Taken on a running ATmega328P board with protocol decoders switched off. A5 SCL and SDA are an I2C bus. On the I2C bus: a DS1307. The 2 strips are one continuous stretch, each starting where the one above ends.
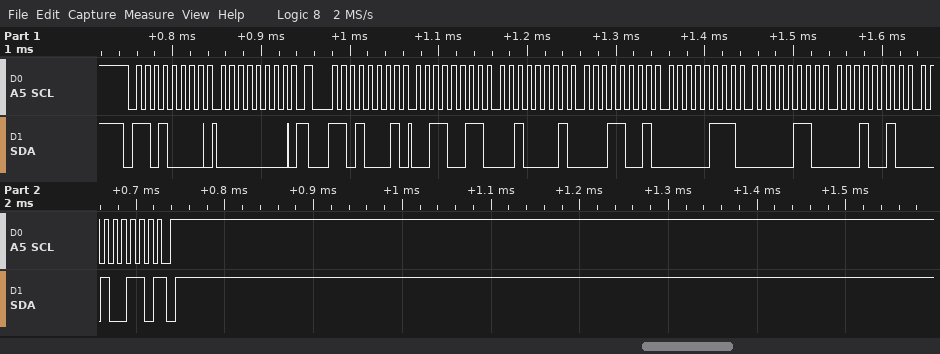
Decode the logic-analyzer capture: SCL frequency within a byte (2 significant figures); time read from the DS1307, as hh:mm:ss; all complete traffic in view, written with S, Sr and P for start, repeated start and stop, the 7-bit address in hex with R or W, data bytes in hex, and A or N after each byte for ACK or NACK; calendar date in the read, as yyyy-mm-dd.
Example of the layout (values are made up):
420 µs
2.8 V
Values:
100 kHz
19:21:33
S 68W A 00 A Sr 68R A 33 A 21 A 19 A 07 A 06 A 12 A 26 N P
2026-12-06
